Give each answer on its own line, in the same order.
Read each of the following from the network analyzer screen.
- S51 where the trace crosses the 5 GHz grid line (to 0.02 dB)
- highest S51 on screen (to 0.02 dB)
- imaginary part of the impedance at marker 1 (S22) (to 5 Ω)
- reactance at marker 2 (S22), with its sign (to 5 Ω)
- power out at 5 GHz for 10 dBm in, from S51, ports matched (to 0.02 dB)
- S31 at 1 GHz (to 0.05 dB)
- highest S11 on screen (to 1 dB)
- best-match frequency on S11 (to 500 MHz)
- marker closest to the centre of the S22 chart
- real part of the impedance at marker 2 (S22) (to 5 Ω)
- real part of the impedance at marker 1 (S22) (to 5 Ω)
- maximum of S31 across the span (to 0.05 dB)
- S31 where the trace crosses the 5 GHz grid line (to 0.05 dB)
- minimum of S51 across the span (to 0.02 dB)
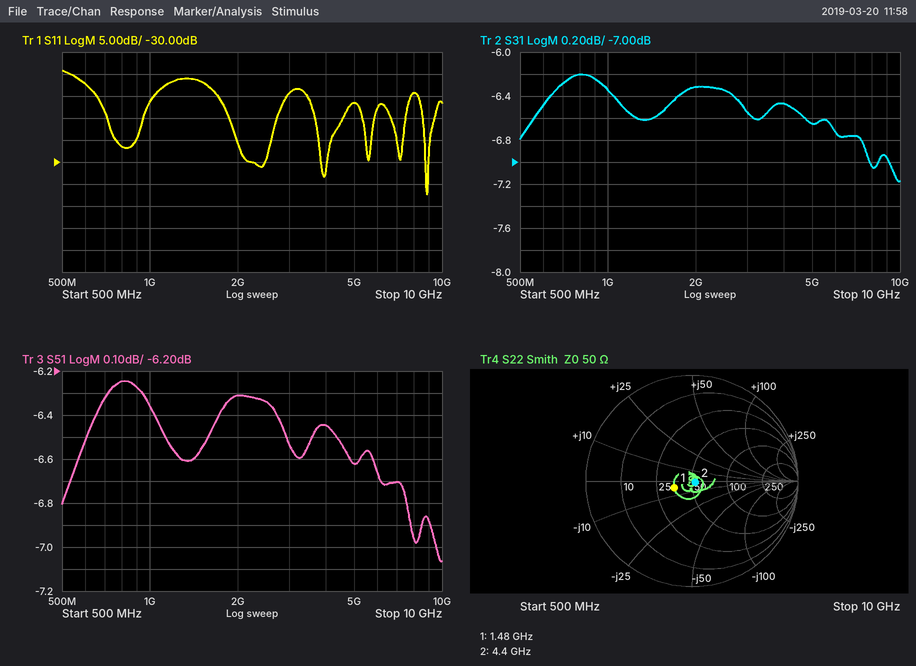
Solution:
-6.62 dB
-6.24 dB
-5 Ω
0 Ω
3.38 dBm
-6.35 dB
-9 dB
9.0 GHz
marker 2
55 Ω
35 Ω
-6.20 dB
-6.65 dB
-7.06 dB
